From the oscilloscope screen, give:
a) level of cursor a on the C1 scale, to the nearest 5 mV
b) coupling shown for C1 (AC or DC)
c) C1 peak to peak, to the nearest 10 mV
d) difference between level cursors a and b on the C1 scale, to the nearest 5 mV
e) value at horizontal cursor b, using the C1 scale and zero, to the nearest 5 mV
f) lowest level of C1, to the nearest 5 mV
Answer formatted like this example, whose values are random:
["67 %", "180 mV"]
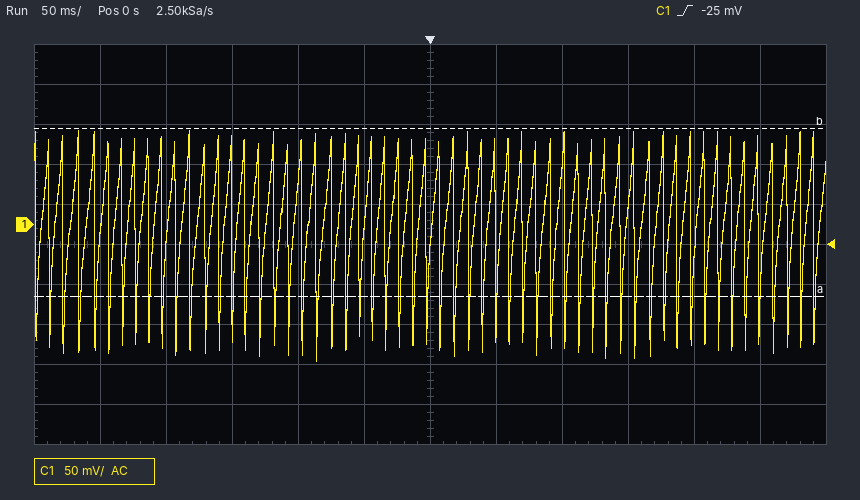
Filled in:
["-90 mV", "AC", "290 mV", "210 mV", "120 mV", "-170 mV"]
